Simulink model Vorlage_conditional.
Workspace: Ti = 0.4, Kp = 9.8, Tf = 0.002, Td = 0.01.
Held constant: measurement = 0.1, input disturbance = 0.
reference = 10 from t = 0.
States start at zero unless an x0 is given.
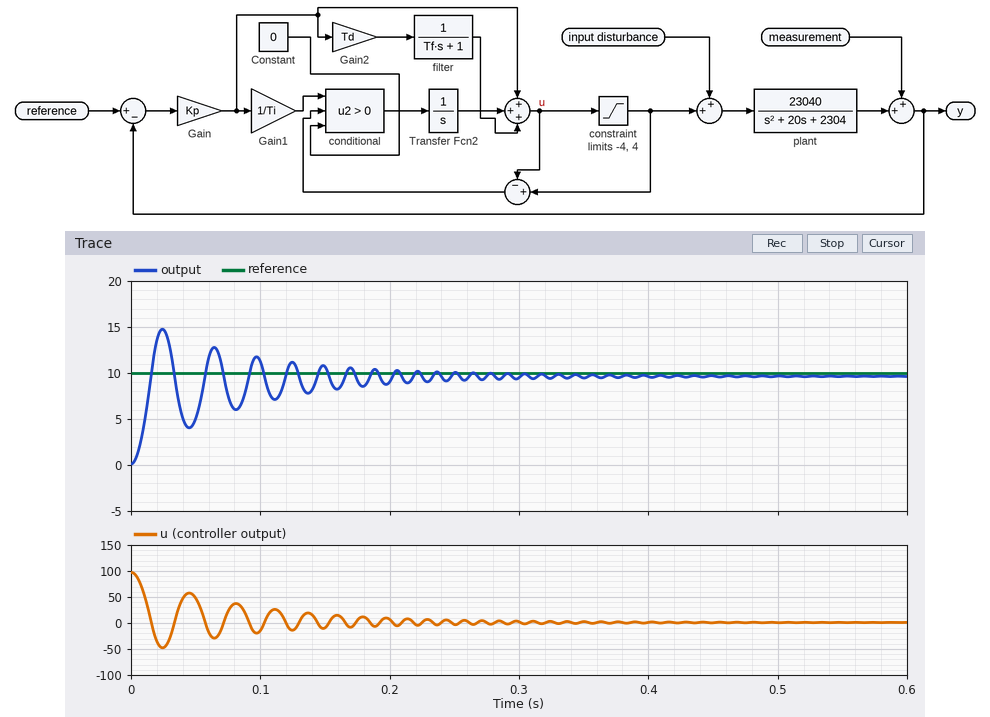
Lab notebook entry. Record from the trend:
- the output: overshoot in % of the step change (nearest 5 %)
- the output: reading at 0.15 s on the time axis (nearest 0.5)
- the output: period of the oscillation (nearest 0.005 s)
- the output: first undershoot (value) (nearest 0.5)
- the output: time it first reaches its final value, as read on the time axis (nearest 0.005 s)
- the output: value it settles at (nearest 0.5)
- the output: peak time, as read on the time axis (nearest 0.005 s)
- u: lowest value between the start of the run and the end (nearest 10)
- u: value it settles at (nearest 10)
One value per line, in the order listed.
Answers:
55 %
10.5
0.040 s
4.0
0.015 s
9.5
0.025 s
-50
0
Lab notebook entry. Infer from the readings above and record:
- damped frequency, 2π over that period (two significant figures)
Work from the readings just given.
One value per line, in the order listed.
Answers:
160 rad/s
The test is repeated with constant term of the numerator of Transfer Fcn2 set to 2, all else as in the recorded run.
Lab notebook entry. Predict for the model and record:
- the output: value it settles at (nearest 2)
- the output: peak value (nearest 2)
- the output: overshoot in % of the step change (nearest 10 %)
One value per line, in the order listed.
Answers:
10
14
60 %
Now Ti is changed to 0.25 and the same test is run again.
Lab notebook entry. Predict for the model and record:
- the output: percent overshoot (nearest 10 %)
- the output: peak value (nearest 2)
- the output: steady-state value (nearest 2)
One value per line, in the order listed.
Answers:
60 %
14
10
